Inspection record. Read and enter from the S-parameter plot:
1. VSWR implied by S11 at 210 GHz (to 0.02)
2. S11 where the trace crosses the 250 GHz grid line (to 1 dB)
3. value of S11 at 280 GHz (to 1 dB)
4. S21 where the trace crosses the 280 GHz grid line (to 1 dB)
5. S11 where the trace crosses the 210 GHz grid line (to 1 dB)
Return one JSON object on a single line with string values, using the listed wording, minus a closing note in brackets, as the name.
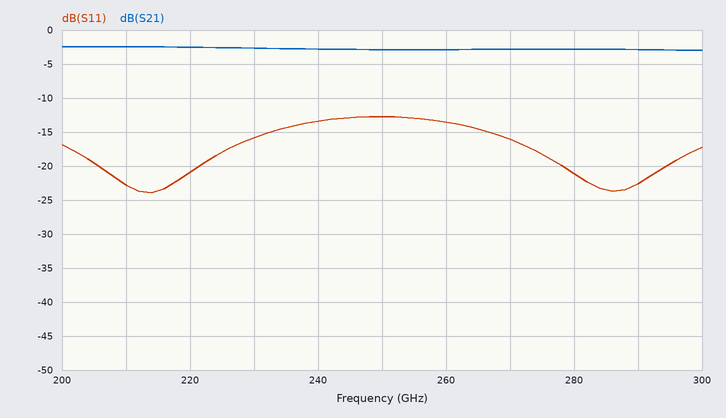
{"VSWR implied by S11 at 210 GHz": "1.16", "S11 where the trace crosses the 250 GHz grid line": "-13 dB", "value of S11 at 280 GHz": "-21 dB", "S21 where the trace crosses the 280 GHz grid line": "-3 dB", "S11 where the trace crosses the 210 GHz grid line": "-23 dB"}
